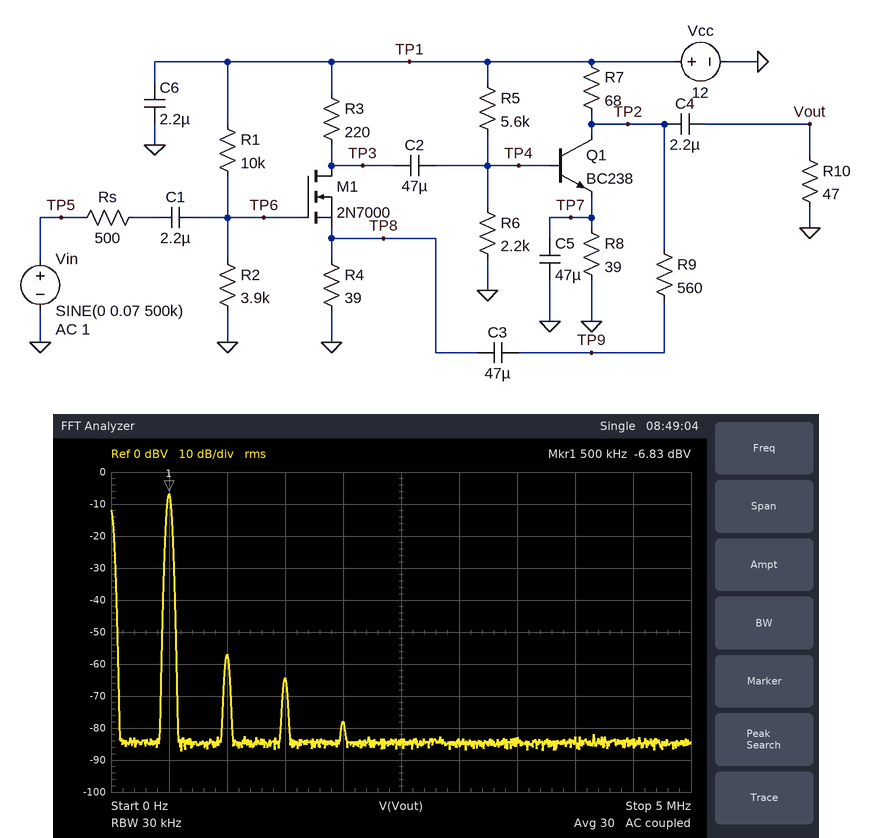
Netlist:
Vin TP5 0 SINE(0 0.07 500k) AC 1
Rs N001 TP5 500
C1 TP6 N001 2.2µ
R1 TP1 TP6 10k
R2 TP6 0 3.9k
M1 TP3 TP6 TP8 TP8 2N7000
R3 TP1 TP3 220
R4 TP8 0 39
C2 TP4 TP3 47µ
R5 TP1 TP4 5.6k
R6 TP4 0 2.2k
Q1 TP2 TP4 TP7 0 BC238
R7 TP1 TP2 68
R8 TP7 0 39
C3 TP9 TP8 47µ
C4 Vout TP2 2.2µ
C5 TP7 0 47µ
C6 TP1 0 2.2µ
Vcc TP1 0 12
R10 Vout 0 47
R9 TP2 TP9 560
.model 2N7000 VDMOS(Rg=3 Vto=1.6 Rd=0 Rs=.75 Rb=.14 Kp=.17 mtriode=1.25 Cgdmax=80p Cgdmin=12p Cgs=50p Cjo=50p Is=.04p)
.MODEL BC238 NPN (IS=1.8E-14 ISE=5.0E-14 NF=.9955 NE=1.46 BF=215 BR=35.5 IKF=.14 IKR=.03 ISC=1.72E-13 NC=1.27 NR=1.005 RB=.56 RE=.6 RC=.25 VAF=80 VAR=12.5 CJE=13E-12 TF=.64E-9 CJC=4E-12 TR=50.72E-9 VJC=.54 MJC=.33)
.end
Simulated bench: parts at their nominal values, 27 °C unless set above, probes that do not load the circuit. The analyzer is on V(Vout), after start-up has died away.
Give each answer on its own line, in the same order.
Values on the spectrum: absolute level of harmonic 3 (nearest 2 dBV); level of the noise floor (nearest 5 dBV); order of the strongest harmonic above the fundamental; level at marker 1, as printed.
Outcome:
-64 dBV
-85 dBV
2
-6.83 dBV
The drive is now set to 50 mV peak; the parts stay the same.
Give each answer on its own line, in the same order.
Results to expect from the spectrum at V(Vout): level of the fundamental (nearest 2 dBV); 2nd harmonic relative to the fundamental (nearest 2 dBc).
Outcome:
-10 dBV
-52 dBc
